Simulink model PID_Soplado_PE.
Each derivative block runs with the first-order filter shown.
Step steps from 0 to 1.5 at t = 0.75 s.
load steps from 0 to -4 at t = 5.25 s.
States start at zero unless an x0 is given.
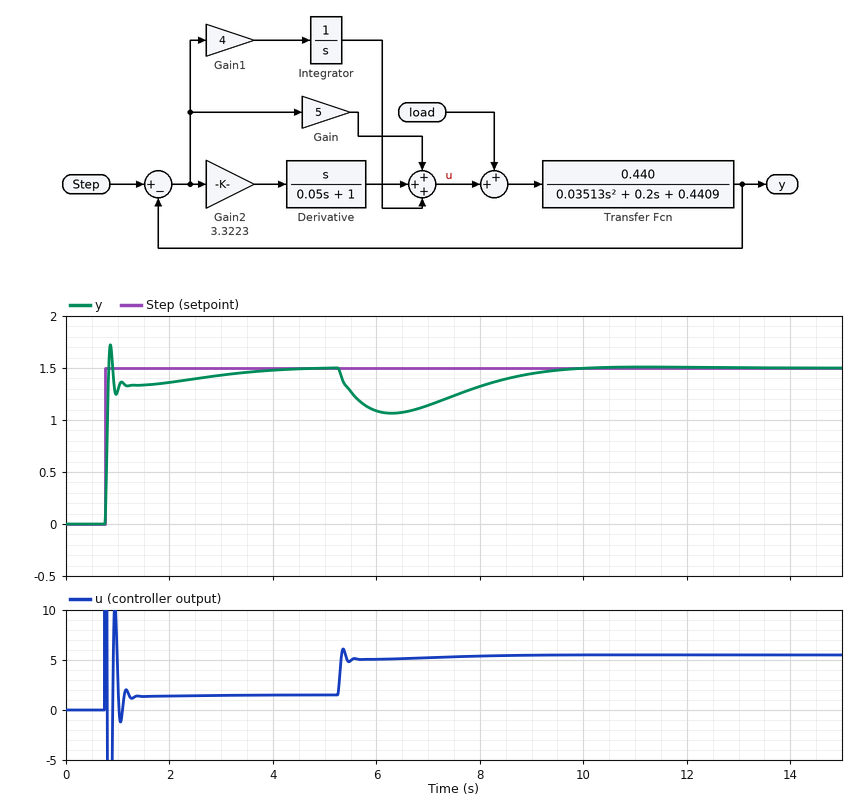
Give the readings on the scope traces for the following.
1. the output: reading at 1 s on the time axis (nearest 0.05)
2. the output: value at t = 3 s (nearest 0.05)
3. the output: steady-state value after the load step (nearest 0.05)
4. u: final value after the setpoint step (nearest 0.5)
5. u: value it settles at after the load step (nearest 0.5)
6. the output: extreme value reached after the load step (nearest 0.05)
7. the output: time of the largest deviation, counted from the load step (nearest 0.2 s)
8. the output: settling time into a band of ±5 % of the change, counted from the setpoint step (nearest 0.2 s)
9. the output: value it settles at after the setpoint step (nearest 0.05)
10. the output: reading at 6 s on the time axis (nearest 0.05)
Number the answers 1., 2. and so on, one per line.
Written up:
1. 1.30
2. 1.45
3. 1.50
4. 1.5
5. 5.5
6. 1.05
7. 1.0 s
8. 2.2 s
9. 1.50
10. 1.10
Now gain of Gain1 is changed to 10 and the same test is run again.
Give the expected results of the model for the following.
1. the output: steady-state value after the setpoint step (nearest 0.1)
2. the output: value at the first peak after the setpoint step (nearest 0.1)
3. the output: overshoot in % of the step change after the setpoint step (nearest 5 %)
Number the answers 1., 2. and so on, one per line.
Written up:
1. 1.5
2. 1.7
3. 15 %
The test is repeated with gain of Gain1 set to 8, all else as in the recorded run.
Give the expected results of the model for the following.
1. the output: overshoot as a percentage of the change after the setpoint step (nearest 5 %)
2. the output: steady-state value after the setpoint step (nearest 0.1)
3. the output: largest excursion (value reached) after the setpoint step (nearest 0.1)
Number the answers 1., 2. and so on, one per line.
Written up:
1. 15 %
2. 1.5
3. 1.7
